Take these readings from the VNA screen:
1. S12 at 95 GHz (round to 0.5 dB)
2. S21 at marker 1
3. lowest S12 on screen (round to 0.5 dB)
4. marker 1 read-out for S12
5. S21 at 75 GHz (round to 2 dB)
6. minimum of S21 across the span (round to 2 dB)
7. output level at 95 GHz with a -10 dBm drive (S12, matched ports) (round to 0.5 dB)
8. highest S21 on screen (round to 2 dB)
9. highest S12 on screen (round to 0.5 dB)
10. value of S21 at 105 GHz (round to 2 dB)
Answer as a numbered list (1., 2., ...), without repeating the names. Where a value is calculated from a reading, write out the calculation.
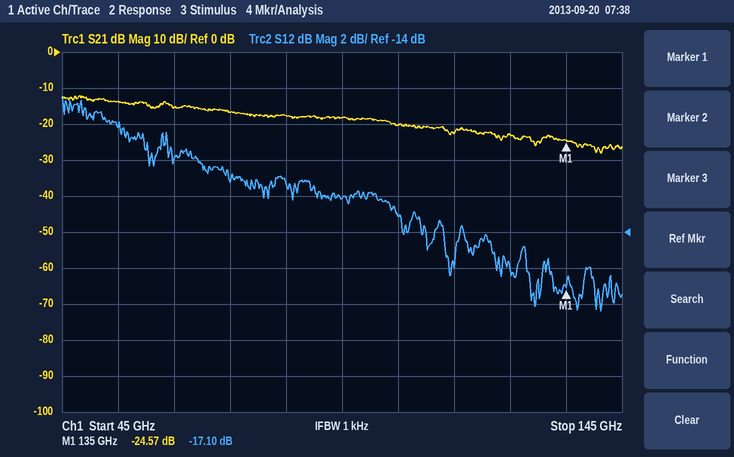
1. -12.0 dB
2. -24.57 dB
3. -18.5 dB
4. -17.10 dB
5. -16 dB
6. -28 dB
7. -10 dBm + (-12.0 dB) = -22.0 dBm
8. -12 dB
9. -6.5 dB
10. -20 dB
